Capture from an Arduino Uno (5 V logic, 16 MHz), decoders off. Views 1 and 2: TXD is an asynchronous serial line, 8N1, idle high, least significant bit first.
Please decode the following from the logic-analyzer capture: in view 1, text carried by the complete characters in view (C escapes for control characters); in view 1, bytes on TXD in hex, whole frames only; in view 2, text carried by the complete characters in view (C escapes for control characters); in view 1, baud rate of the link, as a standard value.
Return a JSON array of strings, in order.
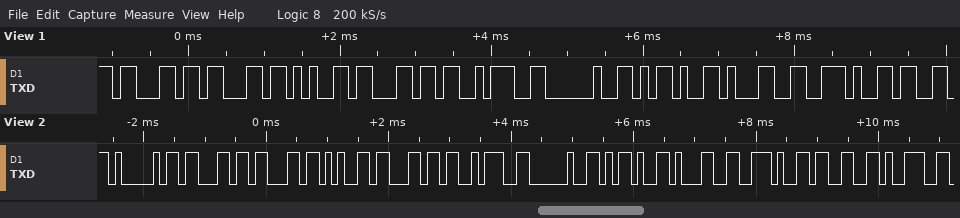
["\"ccel: -1.\"", "63 63 65 6C 3A 20 2D 31 2E", "\"Accel: -1.39\"", "9600 baud"]
